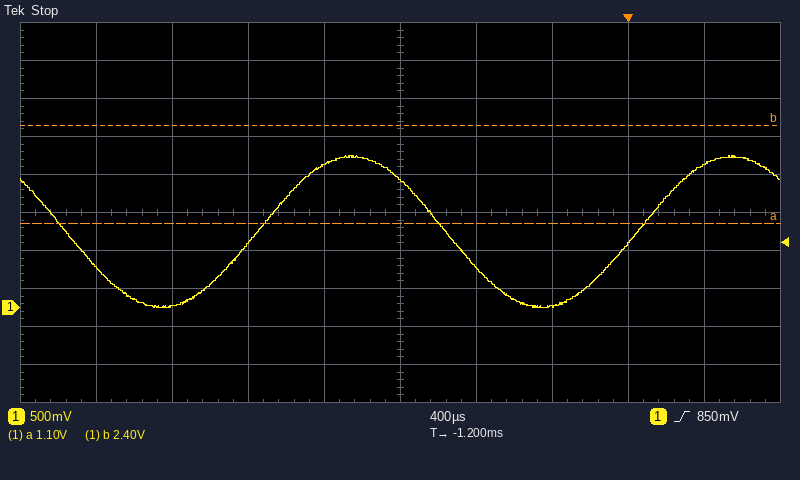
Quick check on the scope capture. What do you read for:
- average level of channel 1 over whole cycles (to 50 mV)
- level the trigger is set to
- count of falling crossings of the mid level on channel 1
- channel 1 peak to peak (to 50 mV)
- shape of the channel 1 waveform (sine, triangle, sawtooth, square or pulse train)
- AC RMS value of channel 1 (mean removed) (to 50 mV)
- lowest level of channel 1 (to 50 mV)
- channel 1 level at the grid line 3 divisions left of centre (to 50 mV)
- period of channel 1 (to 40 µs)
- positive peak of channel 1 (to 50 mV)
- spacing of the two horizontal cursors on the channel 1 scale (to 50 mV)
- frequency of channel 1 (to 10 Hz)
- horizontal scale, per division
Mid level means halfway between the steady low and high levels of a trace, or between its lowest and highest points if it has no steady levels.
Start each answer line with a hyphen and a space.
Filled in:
- 1.00 V
- 850 mV
- 2
- 2.00 V
- sine
- 700 mV
- 0 mV
- 0 mV
- 2.00 ms
- 2.00 V
- 1.30 V
- 500 Hz
- 400 µs
